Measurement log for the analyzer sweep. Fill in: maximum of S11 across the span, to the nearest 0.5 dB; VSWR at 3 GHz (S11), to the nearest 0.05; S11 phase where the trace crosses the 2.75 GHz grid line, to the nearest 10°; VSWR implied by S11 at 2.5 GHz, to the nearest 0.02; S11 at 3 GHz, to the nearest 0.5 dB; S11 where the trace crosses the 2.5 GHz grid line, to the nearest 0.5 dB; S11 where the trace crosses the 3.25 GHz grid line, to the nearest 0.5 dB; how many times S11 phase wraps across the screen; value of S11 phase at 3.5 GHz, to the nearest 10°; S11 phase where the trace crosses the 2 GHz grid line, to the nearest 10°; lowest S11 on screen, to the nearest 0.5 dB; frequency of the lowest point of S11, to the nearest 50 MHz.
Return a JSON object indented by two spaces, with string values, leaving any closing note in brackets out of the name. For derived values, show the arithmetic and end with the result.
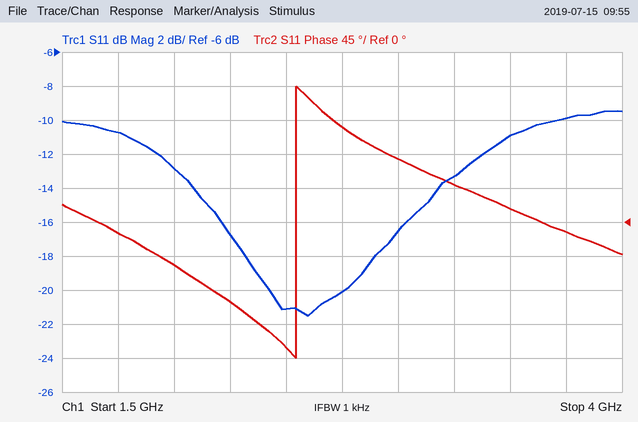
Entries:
{
  "maximum of S11 across the span, to the nearest 0.5 dB": "-9.5 dB",
  "VSWR at 3 GHz (S11), to the nearest 0.05": "|Γ| = 10^(-16.5/20) = 0.1496; VSWR = (1 + 0.1496)/(1 − 0.1496) ≈ 1.35",
  "S11 phase where the trace crosses the 2.75 GHz grid line, to the nearest 10°": "130°",
  "VSWR implied by S11 at 2.5 GHz, to the nearest 0.02": "|Γ| = 10^(-21/20) = 0.0891; VSWR = (1 + 0.0891)/(1 − 0.0891) ≈ 1.20",
  "S11 at 3 GHz, to the nearest 0.5 dB": "-16.5 dB",
  "S11 where the trace crosses the 2.5 GHz grid line, to the nearest 0.5 dB": "-21.0 dB",
  "S11 where the trace crosses the 3.25 GHz grid line, to the nearest 0.5 dB": "-13.5 dB",
  "how many times S11 phase wraps across the screen": "1",
  "value of S11 phase at 3.5 GHz, to the nearest 10°": "20°",
  "S11 phase where the trace crosses the 2 GHz grid line, to the nearest 10°": "-60°",
  "lowest S11 on screen, to the nearest 0.5 dB": "-21.5 dB",
  "frequency of the lowest point of S11, to the nearest 50 MHz": "2.60 GHz"
}
